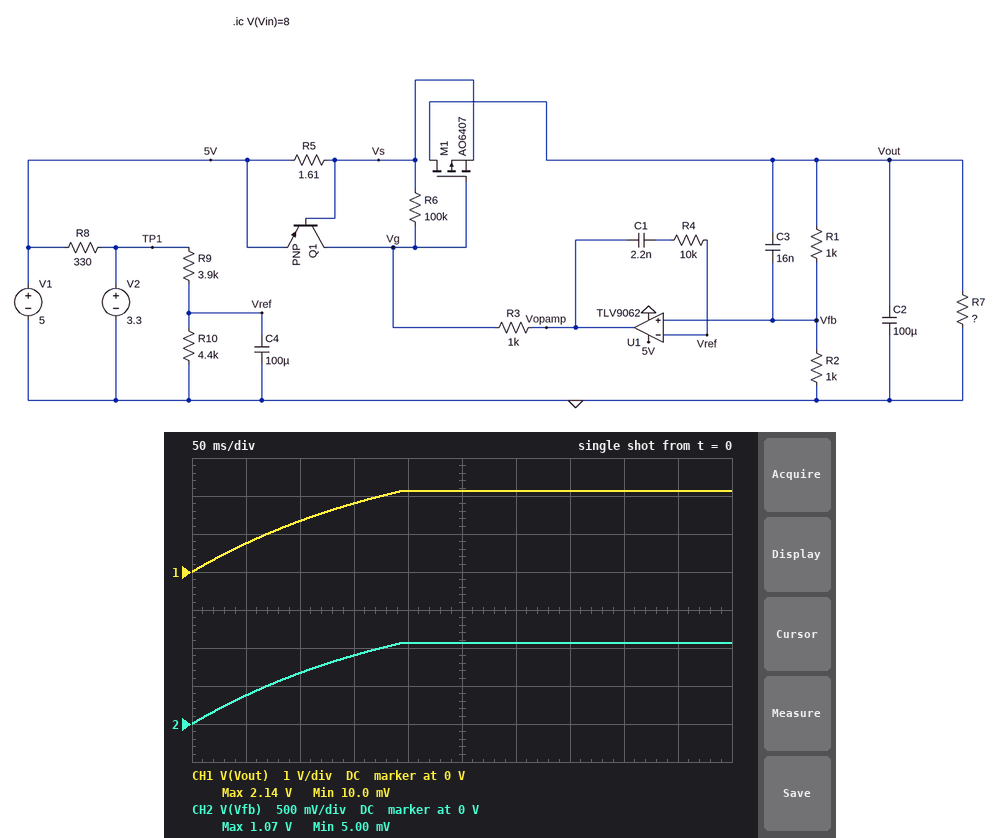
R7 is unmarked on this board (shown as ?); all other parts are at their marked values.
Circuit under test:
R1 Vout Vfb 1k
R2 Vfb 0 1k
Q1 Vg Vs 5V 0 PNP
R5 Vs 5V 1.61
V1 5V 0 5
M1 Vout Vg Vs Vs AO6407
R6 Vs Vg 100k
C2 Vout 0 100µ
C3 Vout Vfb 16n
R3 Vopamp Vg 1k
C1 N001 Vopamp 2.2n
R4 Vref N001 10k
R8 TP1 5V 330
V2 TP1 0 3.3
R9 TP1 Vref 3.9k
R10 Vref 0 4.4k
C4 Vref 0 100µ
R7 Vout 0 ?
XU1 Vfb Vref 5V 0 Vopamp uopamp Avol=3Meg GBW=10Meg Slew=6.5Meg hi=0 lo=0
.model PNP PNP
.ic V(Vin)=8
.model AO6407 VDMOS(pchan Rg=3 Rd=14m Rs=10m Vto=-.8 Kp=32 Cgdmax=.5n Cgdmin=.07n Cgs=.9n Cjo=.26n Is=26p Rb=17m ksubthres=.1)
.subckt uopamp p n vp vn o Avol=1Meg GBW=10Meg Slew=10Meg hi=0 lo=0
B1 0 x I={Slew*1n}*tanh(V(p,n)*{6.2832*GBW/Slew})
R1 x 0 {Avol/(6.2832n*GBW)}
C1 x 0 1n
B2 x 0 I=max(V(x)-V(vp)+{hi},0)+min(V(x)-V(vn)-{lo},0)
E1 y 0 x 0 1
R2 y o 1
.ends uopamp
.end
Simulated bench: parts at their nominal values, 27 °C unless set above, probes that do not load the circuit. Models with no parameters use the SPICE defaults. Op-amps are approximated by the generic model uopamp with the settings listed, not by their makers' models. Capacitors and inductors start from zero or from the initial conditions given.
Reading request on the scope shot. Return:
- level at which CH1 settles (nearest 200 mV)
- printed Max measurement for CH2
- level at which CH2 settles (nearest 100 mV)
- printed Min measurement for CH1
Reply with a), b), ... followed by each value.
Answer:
a) 2.2 V
b) 1.07 V
c) 1.1 V
d) 10.0 mV
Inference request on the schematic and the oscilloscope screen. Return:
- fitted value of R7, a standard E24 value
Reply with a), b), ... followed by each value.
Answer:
a) 4.3 Ω
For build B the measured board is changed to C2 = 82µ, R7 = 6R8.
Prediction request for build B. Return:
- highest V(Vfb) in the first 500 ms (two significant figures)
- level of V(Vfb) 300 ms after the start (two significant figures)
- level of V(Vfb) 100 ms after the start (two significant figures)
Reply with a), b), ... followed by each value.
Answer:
a) 1.6 V
b) 1.3 V
c) 670 mV
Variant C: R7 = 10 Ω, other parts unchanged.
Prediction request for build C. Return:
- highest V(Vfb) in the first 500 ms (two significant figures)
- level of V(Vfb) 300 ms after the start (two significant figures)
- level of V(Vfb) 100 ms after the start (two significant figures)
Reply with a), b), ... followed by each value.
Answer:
a) 1.6 V
b) 1.3 V
c) 670 mV
